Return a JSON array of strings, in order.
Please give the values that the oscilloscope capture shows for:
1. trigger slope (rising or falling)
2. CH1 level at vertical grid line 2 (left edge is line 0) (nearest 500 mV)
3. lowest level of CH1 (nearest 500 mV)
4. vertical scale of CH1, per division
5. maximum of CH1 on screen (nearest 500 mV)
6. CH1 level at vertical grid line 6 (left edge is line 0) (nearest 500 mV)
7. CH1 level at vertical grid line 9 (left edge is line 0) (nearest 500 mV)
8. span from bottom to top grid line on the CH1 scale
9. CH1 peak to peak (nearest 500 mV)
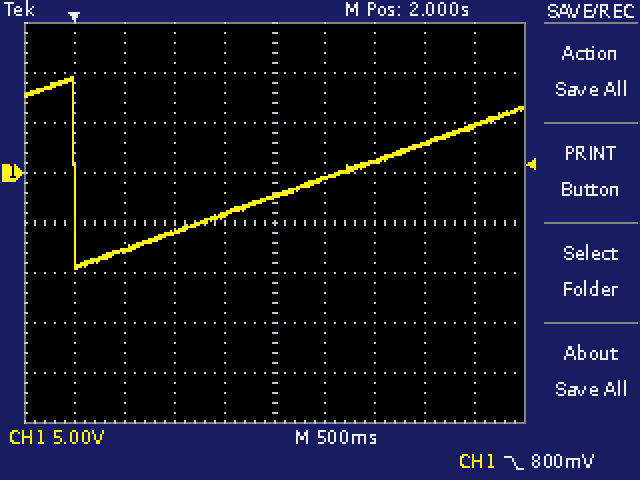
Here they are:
["falling", "-8.0 V", "-9.5 V", "5 V", "9.5 V", "-500 mV", "4.5 V", "40 V", "19.0 V"]
